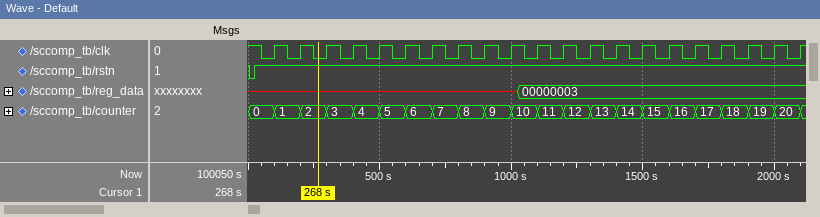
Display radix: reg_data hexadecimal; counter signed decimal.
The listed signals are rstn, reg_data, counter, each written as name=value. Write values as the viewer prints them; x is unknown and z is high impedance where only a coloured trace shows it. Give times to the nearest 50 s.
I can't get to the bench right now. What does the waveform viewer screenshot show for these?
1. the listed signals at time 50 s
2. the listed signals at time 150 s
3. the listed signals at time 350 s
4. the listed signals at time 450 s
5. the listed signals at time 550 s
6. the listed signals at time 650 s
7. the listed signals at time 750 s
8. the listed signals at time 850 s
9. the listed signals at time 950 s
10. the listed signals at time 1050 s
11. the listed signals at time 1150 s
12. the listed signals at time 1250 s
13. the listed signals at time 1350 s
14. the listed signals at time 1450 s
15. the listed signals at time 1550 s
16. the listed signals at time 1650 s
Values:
rstn=1, reg_data=x, counter=0
rstn=1, reg_data=x, counter=1
rstn=1, reg_data=x, counter=3
rstn=1, reg_data=x, counter=4
rstn=1, reg_data=x, counter=5
rstn=1, reg_data=x, counter=6
rstn=1, reg_data=x, counter=7
rstn=1, reg_data=x, counter=8
rstn=1, reg_data=x, counter=9
rstn=1, reg_data=00000003, counter=10
rstn=1, reg_data=00000003, counter=11
rstn=1, reg_data=00000003, counter=12
rstn=1, reg_data=00000003, counter=13
rstn=1, reg_data=00000003, counter=14
rstn=1, reg_data=00000003, counter=15
rstn=1, reg_data=00000003, counter=16
